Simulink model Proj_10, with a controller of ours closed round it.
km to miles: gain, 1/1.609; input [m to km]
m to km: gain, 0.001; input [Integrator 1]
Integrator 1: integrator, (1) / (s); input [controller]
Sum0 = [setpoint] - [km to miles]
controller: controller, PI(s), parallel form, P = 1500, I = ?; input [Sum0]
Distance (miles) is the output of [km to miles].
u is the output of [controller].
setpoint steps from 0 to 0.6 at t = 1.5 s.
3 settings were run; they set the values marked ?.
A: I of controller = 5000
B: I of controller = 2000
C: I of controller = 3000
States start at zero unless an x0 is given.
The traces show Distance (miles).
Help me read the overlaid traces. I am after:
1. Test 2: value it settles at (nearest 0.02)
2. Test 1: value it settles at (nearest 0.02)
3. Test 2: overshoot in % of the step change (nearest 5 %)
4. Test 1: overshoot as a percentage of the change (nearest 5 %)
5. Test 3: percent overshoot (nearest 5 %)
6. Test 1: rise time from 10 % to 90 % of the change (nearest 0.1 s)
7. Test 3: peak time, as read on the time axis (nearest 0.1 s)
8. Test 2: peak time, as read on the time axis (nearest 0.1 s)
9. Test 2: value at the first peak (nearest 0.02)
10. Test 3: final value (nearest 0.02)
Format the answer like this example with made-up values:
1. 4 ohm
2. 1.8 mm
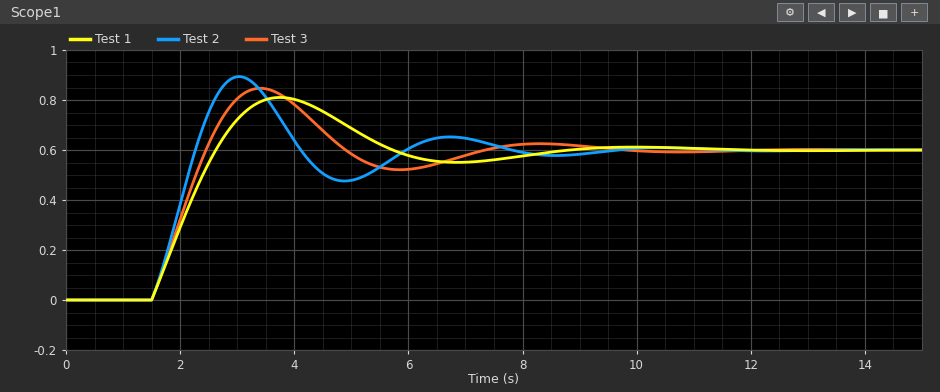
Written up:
1. 0.60
2. 0.60
3. 50 %
4. 35 %
5. 40 %
6. 0.9 s
7. 3.4 s
8. 3.0 s
9. 0.90
10. 0.60
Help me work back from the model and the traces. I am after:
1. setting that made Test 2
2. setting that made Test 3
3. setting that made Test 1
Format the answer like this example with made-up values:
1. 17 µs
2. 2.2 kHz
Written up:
1. A
2. C
3. B
